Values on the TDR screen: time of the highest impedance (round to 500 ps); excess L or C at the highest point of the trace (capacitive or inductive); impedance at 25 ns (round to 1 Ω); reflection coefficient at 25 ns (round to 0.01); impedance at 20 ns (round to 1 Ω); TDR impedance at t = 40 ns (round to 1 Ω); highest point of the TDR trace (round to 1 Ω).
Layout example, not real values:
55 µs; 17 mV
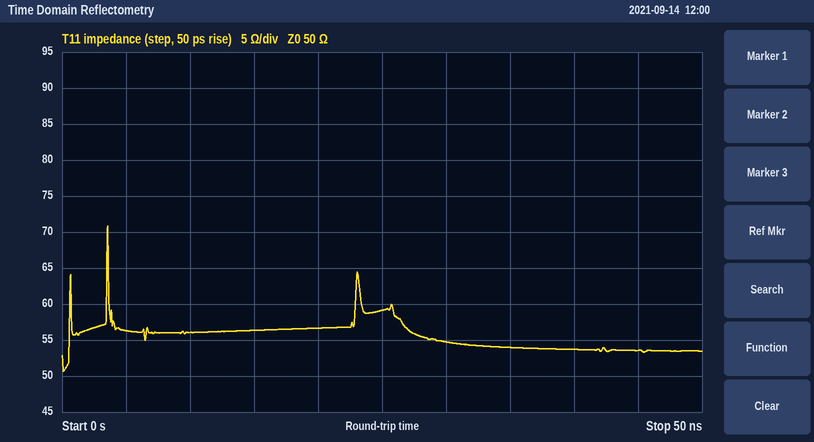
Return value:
3.5 ns; inductive; 59 Ω; +0.08; 57 Ω; 54 Ω; 71 Ω
